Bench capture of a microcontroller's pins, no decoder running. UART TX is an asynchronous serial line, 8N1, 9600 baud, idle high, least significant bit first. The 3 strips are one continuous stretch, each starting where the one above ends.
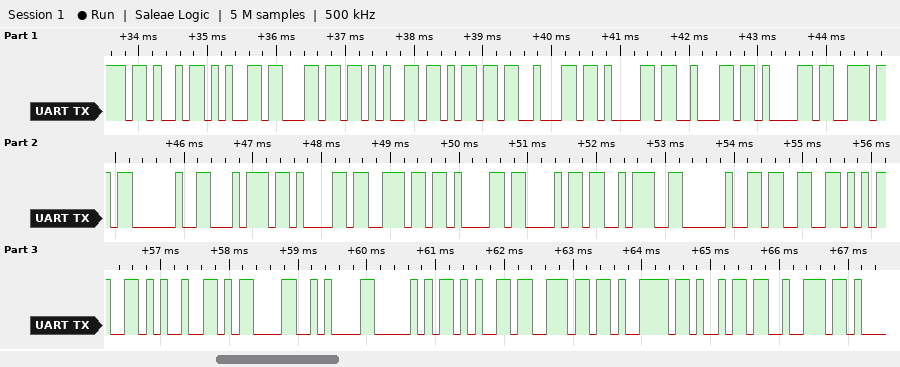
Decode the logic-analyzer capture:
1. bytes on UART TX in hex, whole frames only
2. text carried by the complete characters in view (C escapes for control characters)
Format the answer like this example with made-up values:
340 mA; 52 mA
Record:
0x4B 0x65 0x6C 0x65 0x6D 0x62 0x61 0x62 0x61 0x6E 0x20 0x74 0x61 0x6E 0x61 0x68 0x3A 0x20 0x33 0x35 0x25 0x0D 0x0A 0x50 0x65 0x6E 0x79 0x69 0x72; "Kelembaban tanah: 35%\r\nPenyir"
